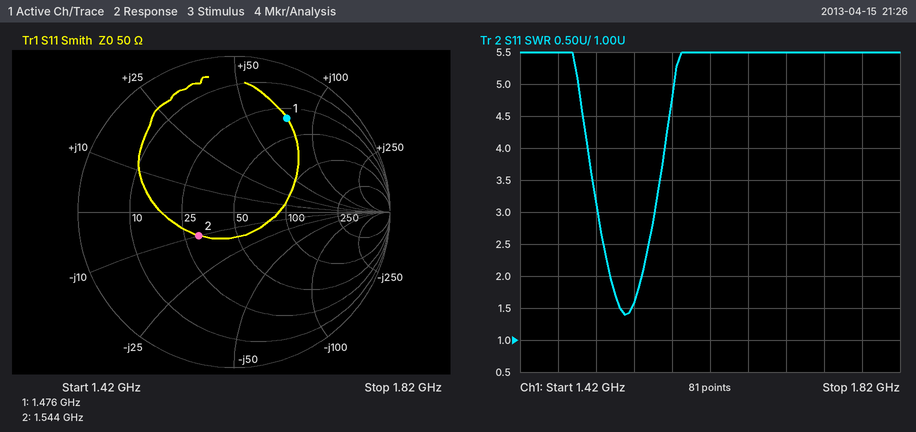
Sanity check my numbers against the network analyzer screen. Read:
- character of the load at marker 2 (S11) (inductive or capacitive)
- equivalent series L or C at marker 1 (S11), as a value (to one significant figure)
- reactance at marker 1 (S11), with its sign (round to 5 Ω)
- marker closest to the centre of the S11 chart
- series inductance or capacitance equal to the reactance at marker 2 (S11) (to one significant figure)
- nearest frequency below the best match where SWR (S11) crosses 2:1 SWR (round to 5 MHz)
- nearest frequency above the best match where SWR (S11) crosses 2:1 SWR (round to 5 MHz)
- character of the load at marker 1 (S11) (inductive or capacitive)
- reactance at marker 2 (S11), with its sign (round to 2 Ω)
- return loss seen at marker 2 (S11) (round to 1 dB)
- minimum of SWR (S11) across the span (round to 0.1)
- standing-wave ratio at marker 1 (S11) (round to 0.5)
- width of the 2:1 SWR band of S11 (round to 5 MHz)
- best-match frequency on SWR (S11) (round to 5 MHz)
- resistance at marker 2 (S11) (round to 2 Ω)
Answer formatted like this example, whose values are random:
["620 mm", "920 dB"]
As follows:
["capacitive", "8 nH", "+75 Ω", "marker 2", "10 pF", "1.515 GHz", "1.550 GHz", "inductive", "-10 Ω", "11 dB", "1.4", "5.5", "35 MHz", "1.530 GHz", "30 Ω"]
